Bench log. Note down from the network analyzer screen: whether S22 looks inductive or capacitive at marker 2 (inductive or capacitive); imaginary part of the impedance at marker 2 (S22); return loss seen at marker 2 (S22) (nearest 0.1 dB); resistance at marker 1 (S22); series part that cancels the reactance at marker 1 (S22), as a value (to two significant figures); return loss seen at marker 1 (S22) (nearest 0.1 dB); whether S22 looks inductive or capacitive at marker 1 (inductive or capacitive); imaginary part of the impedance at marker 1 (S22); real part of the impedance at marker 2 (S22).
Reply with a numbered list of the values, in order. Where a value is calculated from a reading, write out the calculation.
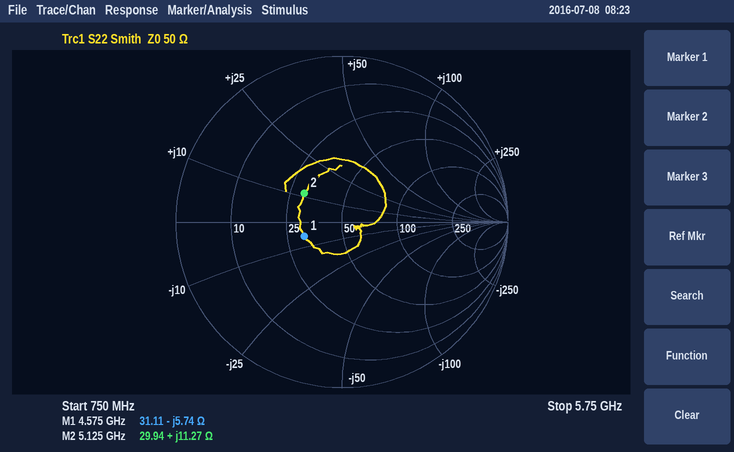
1. inductive
2. +11.27 Ω
3. 10.9 dB
4. 31.11 Ω
5. L = 5.74 Ω/(2π × 4.575 GHz) ≈ 200 pH
6. 12.3 dB
7. capacitive
8. -5.74 Ω
9. 29.94 Ω
